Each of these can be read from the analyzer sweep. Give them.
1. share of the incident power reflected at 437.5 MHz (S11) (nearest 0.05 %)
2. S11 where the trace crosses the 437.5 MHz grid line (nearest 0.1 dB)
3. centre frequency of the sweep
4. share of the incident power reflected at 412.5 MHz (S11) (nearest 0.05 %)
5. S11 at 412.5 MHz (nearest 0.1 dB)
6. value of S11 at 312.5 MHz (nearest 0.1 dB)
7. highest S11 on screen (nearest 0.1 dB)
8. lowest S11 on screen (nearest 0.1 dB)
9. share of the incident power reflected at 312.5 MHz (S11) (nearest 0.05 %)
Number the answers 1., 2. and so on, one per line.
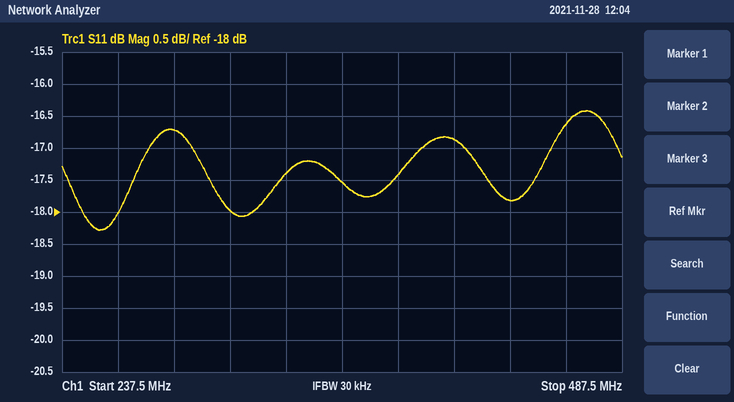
1. 1.65 %
2. -17.8 dB
3. 362.5 MHz
4. 2.05 %
5. -16.9 dB
6. -18.0 dB
7. -16.4 dB
8. -18.3 dB
9. 1.60 %
